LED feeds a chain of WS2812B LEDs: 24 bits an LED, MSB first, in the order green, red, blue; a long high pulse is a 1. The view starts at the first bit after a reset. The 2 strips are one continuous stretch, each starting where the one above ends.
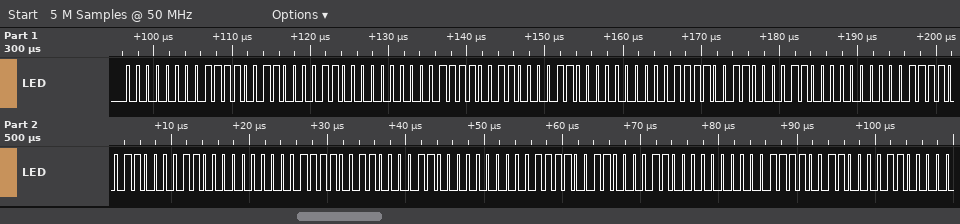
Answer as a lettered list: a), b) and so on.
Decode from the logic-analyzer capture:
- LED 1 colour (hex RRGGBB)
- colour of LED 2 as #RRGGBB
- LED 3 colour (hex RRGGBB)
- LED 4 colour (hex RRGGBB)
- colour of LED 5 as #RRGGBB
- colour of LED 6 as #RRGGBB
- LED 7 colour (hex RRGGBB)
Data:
a) #F3000C
b) #F3000C
c) #F3000C
d) #F3000C
e) #F3000C
f) #F3000C
g) #F3000C
